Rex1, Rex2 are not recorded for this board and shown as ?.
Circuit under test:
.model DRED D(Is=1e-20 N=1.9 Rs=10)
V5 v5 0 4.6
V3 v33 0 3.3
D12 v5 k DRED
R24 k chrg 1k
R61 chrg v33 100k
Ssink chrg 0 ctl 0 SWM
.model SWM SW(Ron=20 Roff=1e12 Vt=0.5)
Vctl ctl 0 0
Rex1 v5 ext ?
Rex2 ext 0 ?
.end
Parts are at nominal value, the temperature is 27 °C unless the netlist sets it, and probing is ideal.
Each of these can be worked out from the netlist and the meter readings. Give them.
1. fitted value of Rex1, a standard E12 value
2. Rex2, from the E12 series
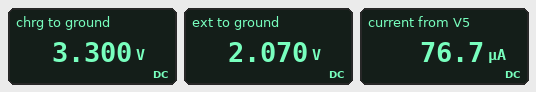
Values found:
33 kΩ
27 kΩ
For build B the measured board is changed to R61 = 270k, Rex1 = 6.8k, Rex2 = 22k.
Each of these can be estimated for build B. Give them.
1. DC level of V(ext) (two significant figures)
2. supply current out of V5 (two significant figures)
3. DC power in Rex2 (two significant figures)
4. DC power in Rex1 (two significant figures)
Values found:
3.5 V
160 µA
560 µW
170 µW
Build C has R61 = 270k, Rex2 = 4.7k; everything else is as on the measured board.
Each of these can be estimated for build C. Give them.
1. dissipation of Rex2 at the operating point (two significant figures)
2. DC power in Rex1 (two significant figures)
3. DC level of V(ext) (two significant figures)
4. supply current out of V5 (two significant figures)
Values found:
70 µW
490 µW
570 mV
120 µA
